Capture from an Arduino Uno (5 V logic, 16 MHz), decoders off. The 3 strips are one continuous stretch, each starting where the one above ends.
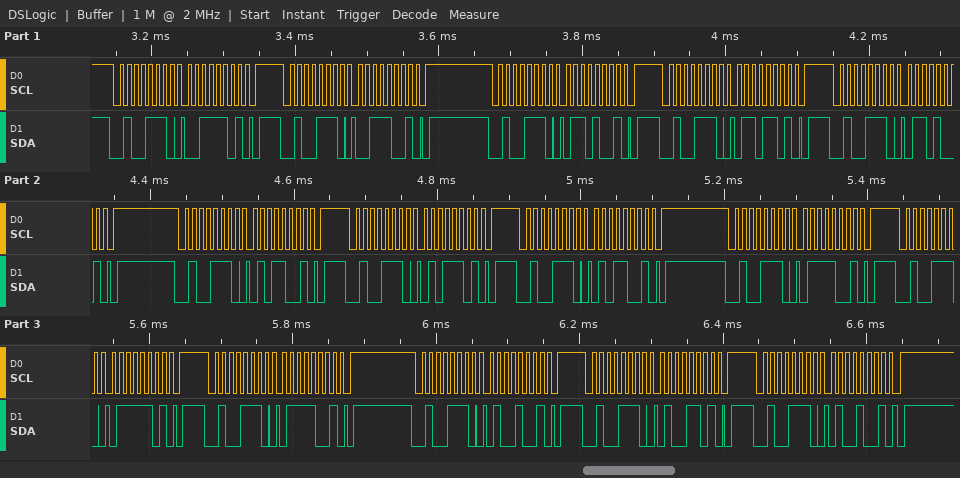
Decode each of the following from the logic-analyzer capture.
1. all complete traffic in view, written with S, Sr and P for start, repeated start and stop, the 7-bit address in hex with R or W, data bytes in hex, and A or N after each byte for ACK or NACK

S 27W A 3D A P S 27W A 39 A P S 27W A 69 A P S 27W A 6D A P S 27W A 69 A P S 27W A 59 A P S 27W A 5D A P S 27W A 59 A P S 27W A 79 A P S 27W A 7D A P S 27W A 79 A P S 27W A 49 A P S 27W A 4D A P S 27W A 49 A P
